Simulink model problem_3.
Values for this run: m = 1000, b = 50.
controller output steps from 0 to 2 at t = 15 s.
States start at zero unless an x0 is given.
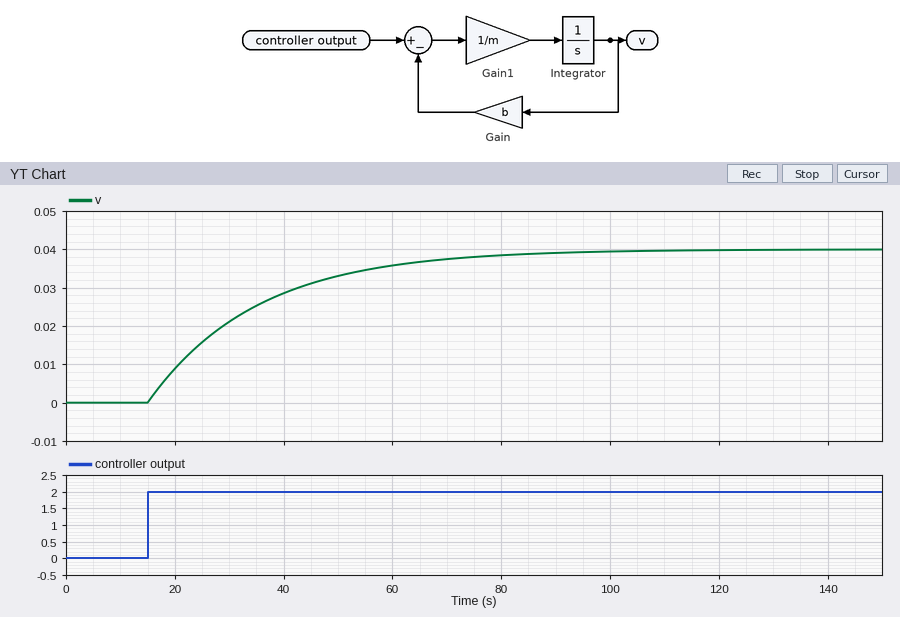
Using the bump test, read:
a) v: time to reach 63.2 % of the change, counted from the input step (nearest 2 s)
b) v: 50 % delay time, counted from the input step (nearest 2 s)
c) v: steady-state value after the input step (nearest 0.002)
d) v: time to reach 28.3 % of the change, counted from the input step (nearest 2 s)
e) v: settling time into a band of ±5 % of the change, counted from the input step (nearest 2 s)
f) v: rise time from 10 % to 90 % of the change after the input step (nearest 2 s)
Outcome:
20 s
14 s
0.040
6 s
60 s
44 s
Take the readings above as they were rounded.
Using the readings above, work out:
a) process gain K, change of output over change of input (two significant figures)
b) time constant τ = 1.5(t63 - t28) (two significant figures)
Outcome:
0.020
21 s
